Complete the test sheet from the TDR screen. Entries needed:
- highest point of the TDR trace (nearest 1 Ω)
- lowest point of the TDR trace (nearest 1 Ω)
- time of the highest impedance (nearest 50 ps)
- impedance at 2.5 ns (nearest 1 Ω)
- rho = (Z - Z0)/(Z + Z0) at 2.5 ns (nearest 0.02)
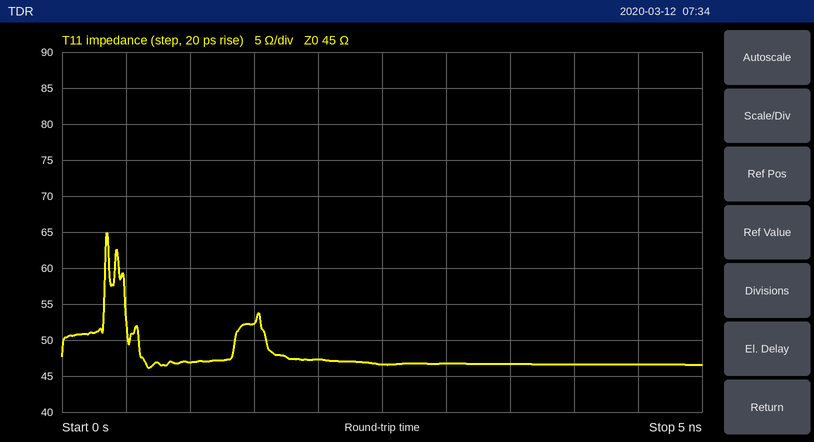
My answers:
65 Ω
46 Ω
350 ps
47 Ω
+0.02
